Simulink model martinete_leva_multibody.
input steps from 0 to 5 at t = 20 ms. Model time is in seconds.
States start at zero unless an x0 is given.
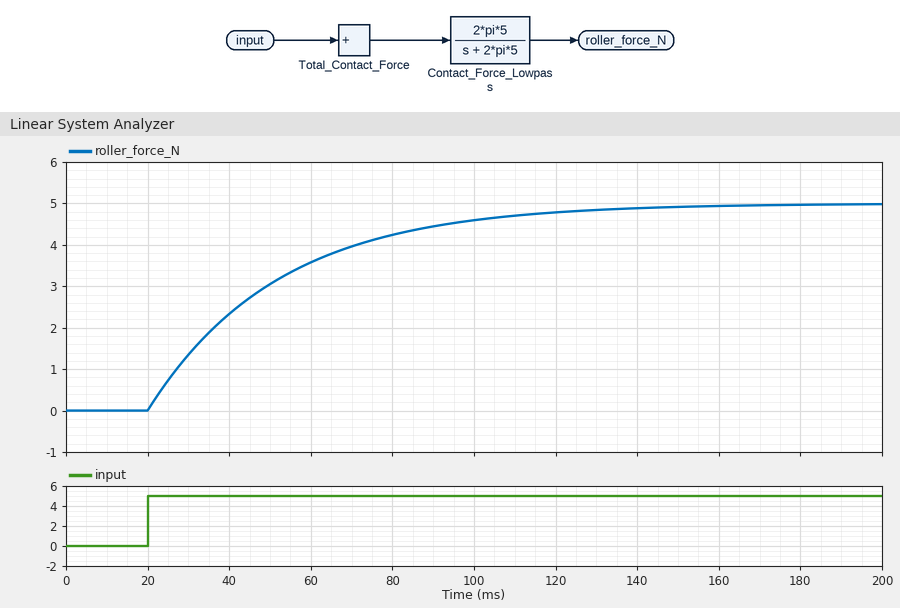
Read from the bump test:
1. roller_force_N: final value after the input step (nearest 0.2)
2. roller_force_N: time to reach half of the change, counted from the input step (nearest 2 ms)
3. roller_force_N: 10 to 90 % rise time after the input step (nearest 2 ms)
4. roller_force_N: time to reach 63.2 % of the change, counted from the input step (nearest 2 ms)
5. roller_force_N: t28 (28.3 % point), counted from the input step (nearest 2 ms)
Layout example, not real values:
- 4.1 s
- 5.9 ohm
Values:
- 5.0
- 22 ms
- 70 ms
- 32 ms
- 10 ms
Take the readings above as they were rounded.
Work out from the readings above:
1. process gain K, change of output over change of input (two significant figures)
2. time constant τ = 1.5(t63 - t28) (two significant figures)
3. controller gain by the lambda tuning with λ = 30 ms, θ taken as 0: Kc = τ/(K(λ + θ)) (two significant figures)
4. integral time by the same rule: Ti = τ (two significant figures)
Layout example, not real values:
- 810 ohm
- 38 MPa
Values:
- 1.0
- 33 ms
- 1.1
- 33 ms
